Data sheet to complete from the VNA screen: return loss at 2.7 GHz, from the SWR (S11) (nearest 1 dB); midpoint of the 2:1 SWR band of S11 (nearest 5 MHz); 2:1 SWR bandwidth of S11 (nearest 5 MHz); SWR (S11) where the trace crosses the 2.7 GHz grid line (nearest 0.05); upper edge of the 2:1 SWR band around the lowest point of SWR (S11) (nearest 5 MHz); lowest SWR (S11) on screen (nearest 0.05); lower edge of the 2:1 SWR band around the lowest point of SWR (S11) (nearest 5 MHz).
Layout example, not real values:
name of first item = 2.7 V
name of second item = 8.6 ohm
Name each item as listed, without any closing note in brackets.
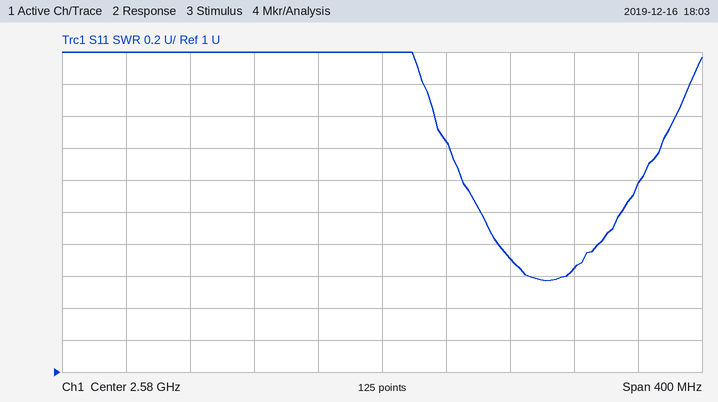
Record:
return loss at 2.7 GHz, from the SWR (S11) = 12 dB
midpoint of the 2:1 SWR band of S11 = 2.685 GHz
2:1 SWR bandwidth of S11 = 90 MHz
SWR (S11) where the trace crosses the 2.7 GHz grid line = 1.65
upper edge of the 2:1 SWR band around the lowest point of SWR (S11) = 2.730 GHz
lowest SWR (S11) on screen = 1.55
lower edge of the 2:1 SWR band around the lowest point of SWR (S11) = 2.640 GHz
